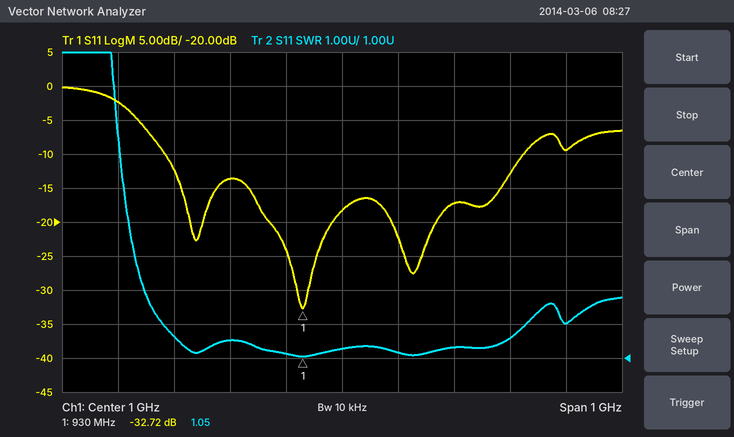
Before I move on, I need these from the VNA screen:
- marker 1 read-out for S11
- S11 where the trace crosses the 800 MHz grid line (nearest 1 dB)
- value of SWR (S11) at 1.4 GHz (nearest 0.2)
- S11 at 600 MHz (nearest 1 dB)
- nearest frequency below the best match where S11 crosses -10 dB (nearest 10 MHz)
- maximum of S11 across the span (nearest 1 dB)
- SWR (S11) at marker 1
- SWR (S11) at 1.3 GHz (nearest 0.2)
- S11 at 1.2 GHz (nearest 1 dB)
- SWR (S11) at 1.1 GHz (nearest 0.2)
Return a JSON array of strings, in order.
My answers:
["-32.72 dB", "-14 dB", "2.0", "-2 dB", "680 MHz", "0 dB", "1.05", "1.6", "-17 dB", "1.2"]
